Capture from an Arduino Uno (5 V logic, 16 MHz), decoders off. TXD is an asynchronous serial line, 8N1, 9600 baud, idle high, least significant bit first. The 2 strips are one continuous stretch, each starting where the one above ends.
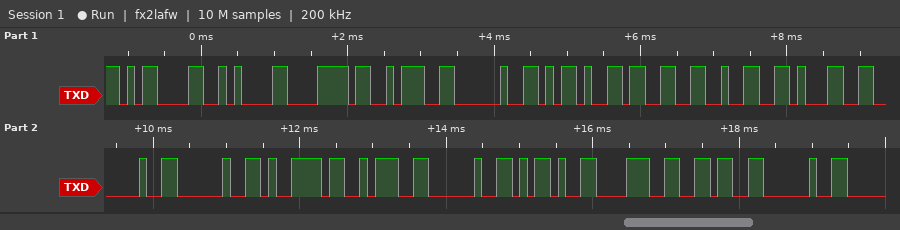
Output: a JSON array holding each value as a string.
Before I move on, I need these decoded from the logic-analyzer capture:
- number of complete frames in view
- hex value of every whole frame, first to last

["18", "0D 0A 78 3A 20 2D 33 32 31 20 20 79 3A 20 2D 38 36 20"]
